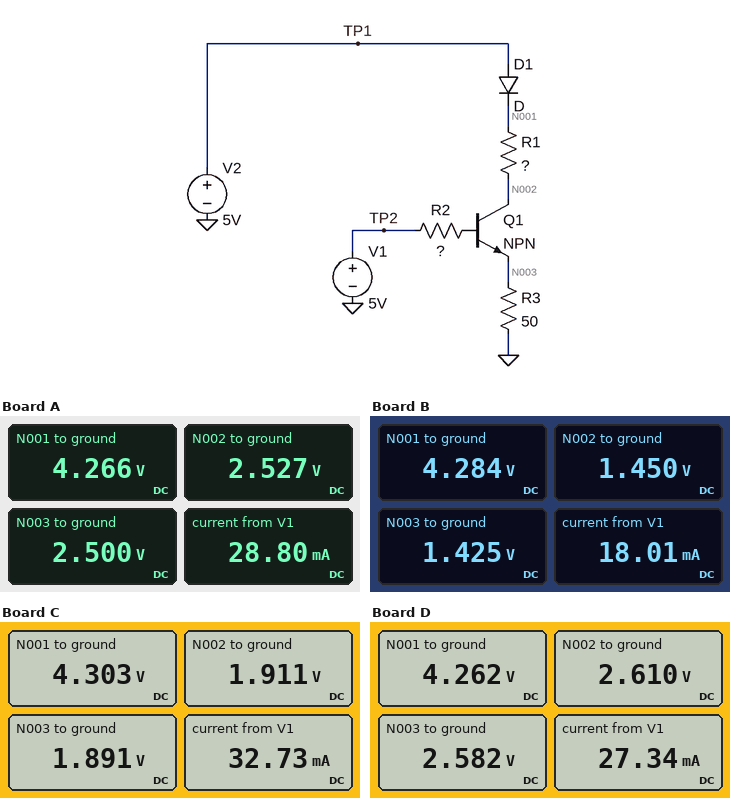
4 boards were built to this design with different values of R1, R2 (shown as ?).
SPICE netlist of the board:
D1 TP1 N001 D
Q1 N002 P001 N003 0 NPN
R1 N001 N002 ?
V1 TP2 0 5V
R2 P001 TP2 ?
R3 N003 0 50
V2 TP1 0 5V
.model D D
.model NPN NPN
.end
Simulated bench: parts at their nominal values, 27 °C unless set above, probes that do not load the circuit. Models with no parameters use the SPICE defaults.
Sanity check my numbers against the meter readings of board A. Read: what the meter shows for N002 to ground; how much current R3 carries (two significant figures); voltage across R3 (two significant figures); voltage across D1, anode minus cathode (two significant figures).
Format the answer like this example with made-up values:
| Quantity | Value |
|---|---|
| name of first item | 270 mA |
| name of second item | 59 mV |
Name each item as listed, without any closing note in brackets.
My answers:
| Quantity | Value |
|---|---|
| what the meter shows for N002 to ground | 2.527 V |
| how much current R3 carries | 50 mA |
| voltage across R3 | 2.5 V |
| voltage across D1, anode minus cathode | 730 mV |
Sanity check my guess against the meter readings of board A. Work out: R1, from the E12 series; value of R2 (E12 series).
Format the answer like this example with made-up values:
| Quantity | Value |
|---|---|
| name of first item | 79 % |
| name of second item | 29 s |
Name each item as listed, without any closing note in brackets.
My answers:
| Quantity | Value |
|---|---|
| R1, from the E12 series | 82 Ω |
| value of R2 | 56 Ω |
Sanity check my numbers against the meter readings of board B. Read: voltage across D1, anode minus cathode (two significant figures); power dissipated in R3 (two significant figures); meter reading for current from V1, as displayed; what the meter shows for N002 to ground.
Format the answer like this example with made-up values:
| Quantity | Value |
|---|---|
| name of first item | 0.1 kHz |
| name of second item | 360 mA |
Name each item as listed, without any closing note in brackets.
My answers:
| Quantity | Value |
|---|---|
| voltage across D1, anode minus cathode | 720 mV |
| power dissipated in R3 | 41 mW |
| meter reading for current from V1, as displayed | 18.01 mA |
| what the meter shows for N002 to ground | 1.450 V |
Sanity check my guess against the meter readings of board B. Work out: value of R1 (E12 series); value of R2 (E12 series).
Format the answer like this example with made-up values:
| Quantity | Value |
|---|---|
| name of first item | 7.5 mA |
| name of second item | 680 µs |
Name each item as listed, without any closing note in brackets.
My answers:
| Quantity | Value |
|---|---|
| value of R1 | 270 Ω |
| value of R2 | 150 Ω |
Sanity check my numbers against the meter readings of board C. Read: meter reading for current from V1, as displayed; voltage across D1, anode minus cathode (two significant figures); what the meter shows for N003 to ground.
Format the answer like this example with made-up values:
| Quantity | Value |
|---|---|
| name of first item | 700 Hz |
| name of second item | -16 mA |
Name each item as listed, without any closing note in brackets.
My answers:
| Quantity | Value |
|---|---|
| meter reading for current from V1, as displayed | 32.73 mA |
| voltage across D1, anode minus cathode | 700 mV |
| what the meter shows for N003 to ground | 1.891 V |
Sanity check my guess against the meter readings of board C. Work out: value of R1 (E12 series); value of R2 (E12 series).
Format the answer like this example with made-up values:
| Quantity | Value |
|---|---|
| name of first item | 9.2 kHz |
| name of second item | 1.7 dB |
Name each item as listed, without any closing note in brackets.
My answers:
| Quantity | Value |
|---|---|
| value of R1 | 470 Ω |
| value of R2 | 68 Ω |
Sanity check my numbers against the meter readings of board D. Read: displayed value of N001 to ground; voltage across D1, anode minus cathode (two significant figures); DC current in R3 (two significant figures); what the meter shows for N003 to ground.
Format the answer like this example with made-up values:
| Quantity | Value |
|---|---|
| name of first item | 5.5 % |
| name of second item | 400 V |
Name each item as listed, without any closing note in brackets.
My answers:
| Quantity | Value |
|---|---|
| displayed value of N001 to ground | 4.262 V |
| voltage across D1, anode minus cathode | 740 mV |
| DC current in R3 | 52 mA |
| what the meter shows for N003 to ground | 2.582 V |
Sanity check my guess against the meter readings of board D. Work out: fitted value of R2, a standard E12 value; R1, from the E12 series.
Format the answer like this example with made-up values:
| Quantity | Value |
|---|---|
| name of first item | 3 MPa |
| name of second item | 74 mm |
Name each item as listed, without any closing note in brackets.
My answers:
| Quantity | Value |
|---|---|
| fitted value of R2, a standard E12 value | 56 Ω |
| R1, from the E12 series | 68 Ω |
